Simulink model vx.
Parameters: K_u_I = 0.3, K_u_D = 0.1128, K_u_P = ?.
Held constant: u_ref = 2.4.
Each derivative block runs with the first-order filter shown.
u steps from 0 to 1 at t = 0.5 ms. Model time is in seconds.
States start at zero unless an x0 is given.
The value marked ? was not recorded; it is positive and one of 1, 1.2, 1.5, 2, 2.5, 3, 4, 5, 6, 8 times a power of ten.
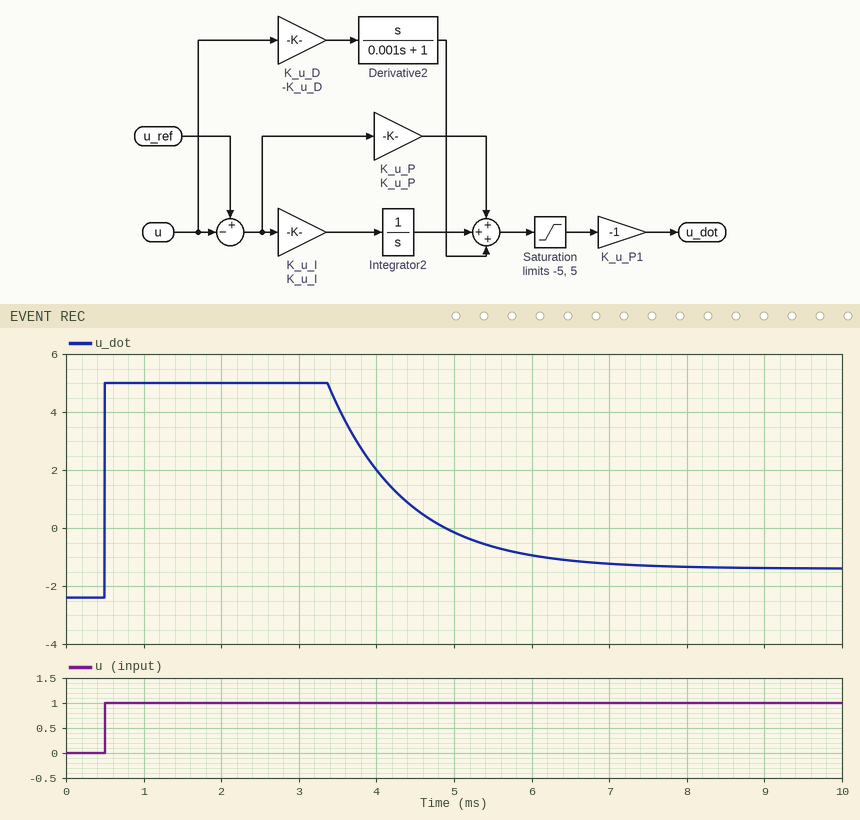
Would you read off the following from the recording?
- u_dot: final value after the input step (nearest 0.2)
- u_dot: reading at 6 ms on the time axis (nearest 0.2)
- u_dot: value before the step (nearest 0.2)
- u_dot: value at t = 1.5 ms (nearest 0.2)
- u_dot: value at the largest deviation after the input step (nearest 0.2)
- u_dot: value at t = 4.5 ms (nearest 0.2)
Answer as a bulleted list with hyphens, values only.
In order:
- -1.4
- -1.0
- -2.4
- 5.0
- 5.0
- 0.6
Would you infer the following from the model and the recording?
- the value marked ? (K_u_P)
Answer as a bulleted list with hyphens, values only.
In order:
- 1
